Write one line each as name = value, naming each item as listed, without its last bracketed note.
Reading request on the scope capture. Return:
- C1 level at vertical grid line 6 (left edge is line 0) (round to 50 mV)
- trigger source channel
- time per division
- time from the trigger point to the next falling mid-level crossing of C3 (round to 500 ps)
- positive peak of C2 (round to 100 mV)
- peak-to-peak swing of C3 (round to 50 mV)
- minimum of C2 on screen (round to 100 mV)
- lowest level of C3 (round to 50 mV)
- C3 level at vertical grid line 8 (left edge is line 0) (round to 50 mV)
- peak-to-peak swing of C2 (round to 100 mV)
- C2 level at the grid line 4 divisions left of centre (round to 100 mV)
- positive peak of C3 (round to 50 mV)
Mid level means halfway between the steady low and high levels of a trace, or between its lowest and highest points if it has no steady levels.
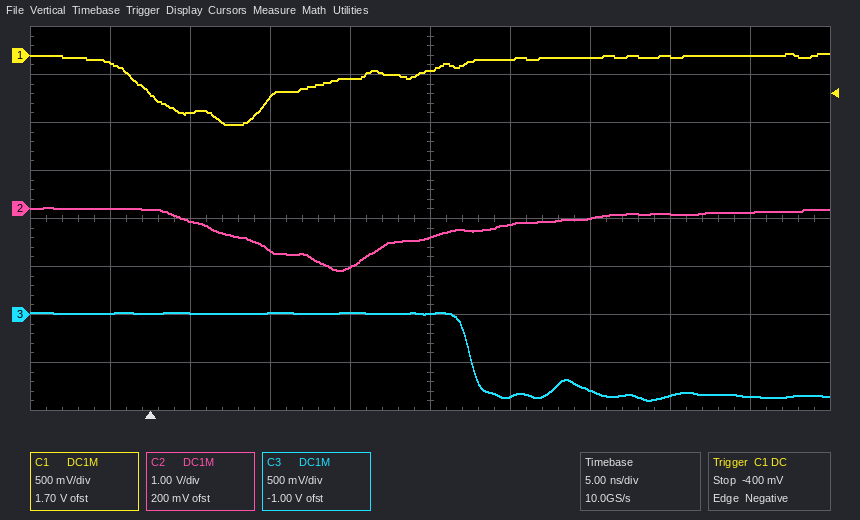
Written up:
C1 level at vertical grid line 6 (left edge is line 0) = -50 mV
trigger source channel = C1
time per division = 5 ns
time from the trigger point to the next falling mid-level crossing of C3 = 20.0 ns
positive peak of C2 = 0.0 V
peak-to-peak swing of C3 = 900 mV
minimum of C2 on screen = -1.3 V
lowest level of C3 = -900 mV
C3 level at vertical grid line 8 (left edge is line 0) = -850 mV
peak-to-peak swing of C2 = 1.3 V
C2 level at the grid line 4 divisions left of centre = 0.0 V
positive peak of C3 = 0 mV
